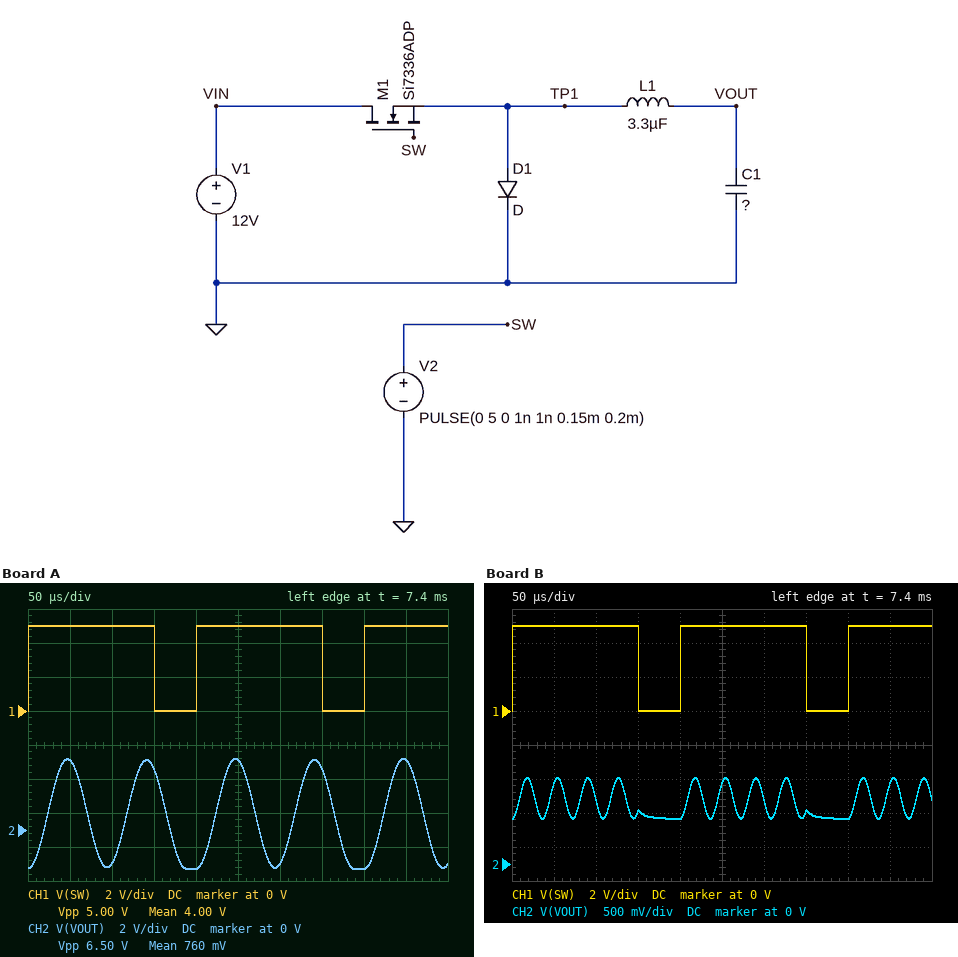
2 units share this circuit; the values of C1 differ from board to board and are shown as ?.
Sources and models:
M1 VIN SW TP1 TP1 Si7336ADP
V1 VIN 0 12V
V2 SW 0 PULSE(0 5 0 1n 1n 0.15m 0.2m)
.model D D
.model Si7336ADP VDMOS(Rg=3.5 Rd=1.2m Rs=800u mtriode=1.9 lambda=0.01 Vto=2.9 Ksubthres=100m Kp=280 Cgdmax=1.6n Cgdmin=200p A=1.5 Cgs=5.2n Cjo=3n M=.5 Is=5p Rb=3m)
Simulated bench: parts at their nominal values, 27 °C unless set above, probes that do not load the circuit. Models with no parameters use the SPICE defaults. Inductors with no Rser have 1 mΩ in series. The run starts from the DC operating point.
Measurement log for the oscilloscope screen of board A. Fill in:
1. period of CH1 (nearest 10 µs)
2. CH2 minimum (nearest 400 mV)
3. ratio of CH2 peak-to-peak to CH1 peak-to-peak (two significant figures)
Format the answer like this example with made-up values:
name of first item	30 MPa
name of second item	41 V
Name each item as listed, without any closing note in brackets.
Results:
period of CH1	200 µs
CH2 minimum	-2.4 V
ratio of CH2 peak-to-peak to CH1 peak-to-peak	1.3
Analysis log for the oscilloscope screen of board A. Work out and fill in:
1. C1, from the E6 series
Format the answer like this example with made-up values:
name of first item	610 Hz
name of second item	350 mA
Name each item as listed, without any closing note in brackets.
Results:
C1, from the E6 series	68 µF
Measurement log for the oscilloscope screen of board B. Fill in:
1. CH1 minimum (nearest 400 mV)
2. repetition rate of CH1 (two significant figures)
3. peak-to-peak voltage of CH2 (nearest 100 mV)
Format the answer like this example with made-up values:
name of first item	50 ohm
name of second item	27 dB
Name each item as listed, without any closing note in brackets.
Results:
CH1 minimum	0 V
repetition rate of CH1	5.0 kHz
peak-to-peak voltage of CH2	600 mV
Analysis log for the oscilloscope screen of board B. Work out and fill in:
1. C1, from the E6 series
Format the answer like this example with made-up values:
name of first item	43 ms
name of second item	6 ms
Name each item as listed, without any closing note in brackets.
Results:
C1, from the E6 series	10 µF
